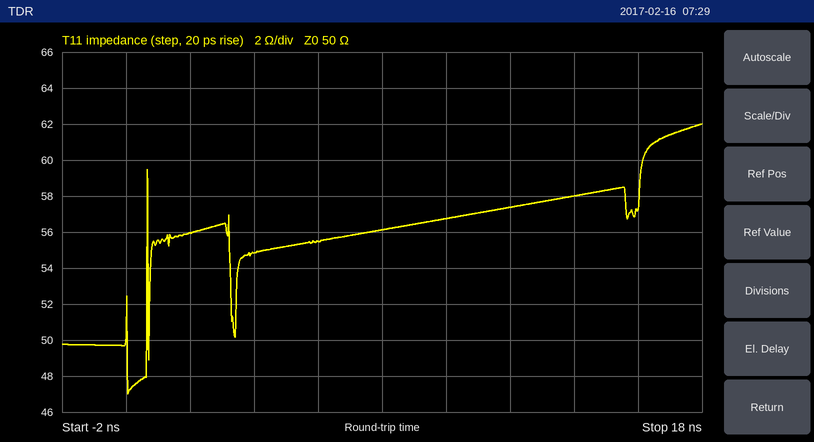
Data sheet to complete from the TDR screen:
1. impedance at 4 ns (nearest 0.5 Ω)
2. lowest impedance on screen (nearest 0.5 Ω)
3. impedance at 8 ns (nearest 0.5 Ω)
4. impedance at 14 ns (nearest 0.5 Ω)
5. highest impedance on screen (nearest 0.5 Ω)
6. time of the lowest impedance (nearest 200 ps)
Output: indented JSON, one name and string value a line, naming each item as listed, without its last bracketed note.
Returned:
{
  "impedance at 4 ns": "55.0 Ω",
  "lowest impedance on screen": "47.0 Ω",
  "impedance at 8 ns": "56.0 Ω",
  "impedance at 14 ns": "58.0 Ω",
  "highest impedance on screen": "62.0 Ω",
  "time of the lowest impedance": "0.0 ns"
}
